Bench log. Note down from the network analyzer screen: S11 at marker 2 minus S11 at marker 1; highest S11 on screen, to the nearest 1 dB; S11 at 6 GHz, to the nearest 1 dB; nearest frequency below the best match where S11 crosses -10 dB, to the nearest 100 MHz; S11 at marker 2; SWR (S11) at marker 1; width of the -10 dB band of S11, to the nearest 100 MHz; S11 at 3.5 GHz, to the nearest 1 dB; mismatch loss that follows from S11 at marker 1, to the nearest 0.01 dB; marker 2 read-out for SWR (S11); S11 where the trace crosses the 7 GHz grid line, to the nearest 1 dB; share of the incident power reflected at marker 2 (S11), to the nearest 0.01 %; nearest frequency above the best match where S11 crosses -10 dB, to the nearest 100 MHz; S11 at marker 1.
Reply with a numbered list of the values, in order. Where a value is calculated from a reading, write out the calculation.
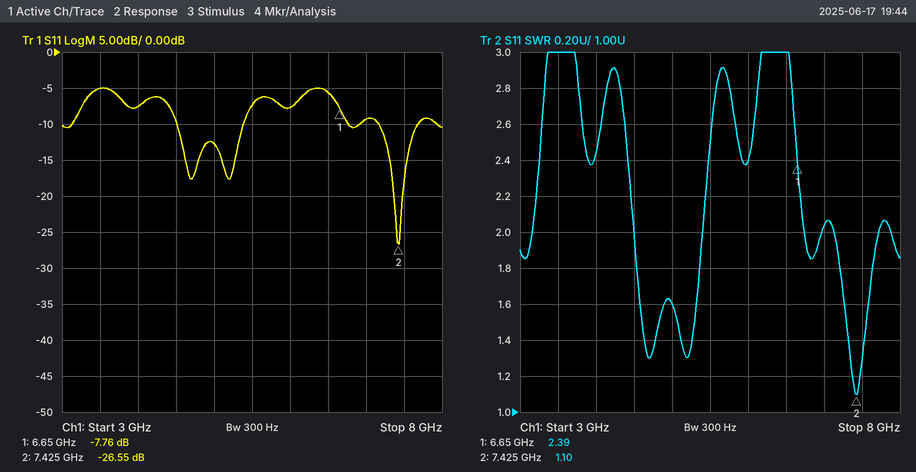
1. -26.55 − (-7.76) = -18.79 dB
2. -5 dB
3. -8 dB
4. 7.2 GHz
5. -26.55 dB
6. 2.39
7. 7.7 GHz − 7.2 GHz = 500 MHz
8. -5 dB
9. −10 log10(1 − 10^(-7.76/10)) ≈ 0.80 dB
10. 1.10
11. -9 dB
12. 10^(-26.55/10) ≈ 0.22 %
13. 7.7 GHz
14. -7.76 dB
